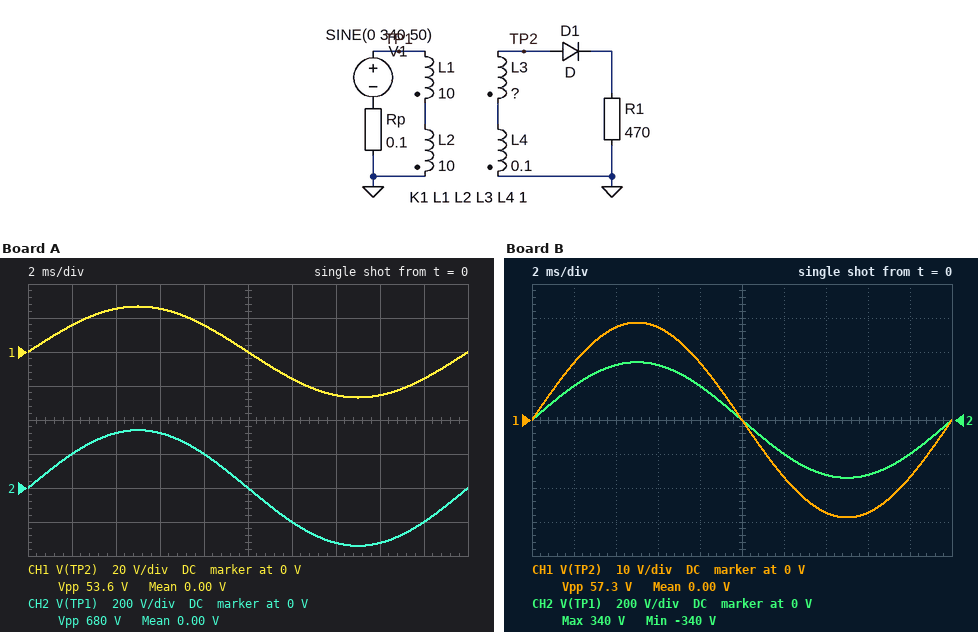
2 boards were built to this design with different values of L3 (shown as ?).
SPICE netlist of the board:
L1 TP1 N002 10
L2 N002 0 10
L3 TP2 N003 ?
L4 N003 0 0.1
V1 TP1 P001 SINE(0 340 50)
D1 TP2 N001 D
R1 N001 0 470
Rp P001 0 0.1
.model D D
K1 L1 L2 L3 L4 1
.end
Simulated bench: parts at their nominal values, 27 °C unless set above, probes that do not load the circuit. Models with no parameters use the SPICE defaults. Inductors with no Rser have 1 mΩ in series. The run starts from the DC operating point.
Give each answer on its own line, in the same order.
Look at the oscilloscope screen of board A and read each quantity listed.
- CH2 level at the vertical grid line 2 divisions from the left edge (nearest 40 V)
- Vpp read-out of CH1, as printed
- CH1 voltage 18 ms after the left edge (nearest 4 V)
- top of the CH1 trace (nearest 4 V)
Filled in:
320 V
53.6 V
-16 V
28 V
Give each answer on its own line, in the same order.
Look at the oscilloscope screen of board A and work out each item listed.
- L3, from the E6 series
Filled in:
33 mH
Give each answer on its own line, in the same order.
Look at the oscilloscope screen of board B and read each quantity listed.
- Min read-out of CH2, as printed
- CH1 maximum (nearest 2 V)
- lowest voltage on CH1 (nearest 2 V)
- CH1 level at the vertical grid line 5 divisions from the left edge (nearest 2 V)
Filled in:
-340 V
28 V
-28 V
0 V
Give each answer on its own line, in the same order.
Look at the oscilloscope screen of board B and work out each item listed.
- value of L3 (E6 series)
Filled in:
47 mH
